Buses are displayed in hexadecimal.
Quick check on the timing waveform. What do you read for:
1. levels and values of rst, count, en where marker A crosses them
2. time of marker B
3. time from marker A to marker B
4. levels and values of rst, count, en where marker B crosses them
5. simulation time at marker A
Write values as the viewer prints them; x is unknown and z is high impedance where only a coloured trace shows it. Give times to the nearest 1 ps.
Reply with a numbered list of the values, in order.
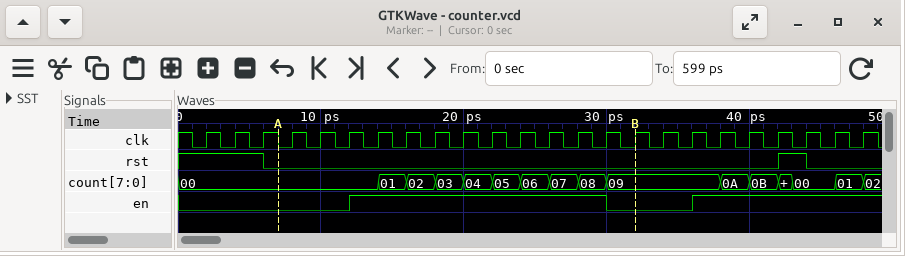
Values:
1. rst=0, count=00, en=0
2. 32 ps
3. 25 ps
4. rst=0, count=09, en=0
5. 7 ps
